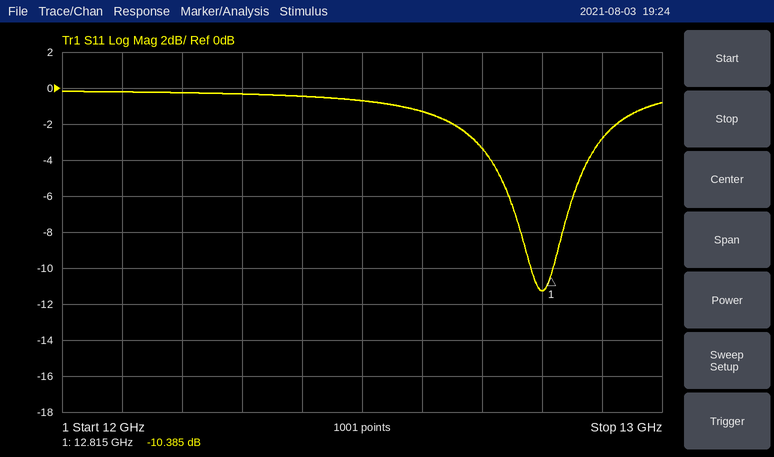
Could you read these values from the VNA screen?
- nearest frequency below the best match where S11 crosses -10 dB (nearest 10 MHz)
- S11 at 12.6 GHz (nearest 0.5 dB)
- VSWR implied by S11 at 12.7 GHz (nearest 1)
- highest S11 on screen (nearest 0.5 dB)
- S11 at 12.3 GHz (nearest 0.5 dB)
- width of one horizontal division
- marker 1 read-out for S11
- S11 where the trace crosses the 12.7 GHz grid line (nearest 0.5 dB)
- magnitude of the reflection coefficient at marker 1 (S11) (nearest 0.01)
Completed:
12.78 GHz
-1.5 dB
5
0.0 dB
-0.5 dB
100 MHz
-10.385 dB
-3.5 dB
0.30
